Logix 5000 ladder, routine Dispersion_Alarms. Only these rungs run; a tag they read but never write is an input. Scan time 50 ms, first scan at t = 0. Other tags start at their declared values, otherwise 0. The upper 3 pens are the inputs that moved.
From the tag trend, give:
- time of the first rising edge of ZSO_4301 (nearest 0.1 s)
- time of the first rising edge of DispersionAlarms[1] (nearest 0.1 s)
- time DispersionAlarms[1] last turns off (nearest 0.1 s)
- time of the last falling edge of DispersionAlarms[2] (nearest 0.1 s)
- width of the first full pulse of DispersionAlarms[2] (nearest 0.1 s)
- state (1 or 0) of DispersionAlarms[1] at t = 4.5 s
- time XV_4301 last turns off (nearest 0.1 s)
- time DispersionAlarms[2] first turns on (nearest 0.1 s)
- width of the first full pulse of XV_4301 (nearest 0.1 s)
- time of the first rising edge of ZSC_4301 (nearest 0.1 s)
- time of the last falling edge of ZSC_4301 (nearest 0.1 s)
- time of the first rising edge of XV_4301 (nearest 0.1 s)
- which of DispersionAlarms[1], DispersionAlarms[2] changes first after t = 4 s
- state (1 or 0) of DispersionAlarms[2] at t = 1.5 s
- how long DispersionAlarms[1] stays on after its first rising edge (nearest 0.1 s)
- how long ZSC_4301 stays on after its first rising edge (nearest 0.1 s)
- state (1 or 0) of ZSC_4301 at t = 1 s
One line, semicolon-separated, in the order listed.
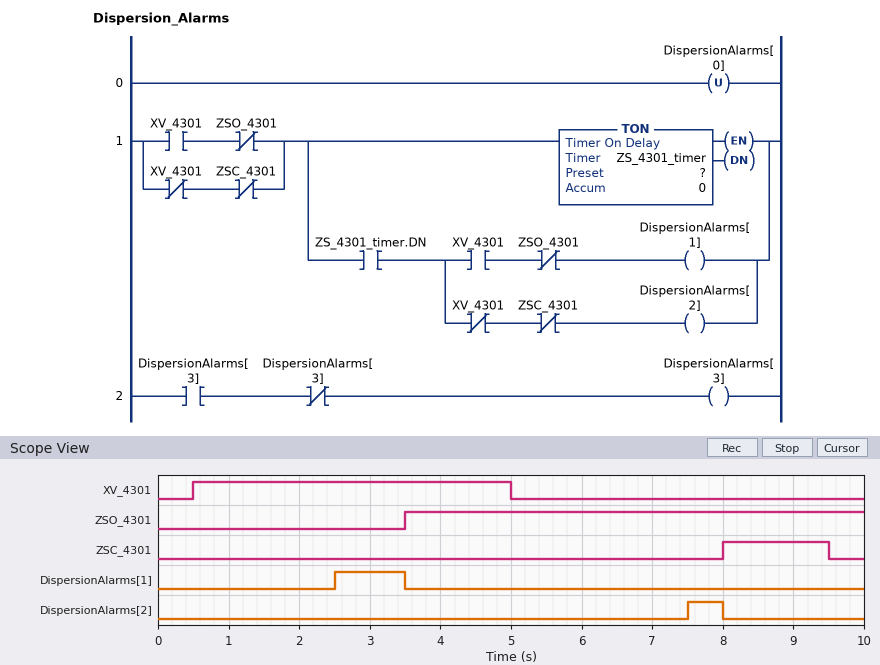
3.5 s; 2.5 s; 3.5 s; 8.0 s; 0.5 s; 0; 5.0 s; 7.5 s; 4.5 s; 8.0 s; 9.5 s; 0.5 s; DispersionAlarms[2]; 0; 1.0 s; 1.5 s; 0
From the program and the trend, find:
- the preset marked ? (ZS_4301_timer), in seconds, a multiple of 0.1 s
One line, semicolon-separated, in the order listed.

2.5 s
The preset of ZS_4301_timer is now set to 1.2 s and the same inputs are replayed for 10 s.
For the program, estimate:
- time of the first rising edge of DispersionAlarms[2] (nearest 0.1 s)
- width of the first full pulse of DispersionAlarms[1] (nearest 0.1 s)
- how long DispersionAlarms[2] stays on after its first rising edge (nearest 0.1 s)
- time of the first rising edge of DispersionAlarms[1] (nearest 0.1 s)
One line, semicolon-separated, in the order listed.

6.2 s; 2.3 s; 1.8 s; 1.2 s
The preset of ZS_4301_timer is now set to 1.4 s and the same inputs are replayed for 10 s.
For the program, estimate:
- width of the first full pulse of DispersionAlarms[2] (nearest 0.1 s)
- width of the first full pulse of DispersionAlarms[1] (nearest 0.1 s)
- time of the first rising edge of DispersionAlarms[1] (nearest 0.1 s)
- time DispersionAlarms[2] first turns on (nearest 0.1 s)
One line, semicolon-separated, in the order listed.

1.6 s; 2.1 s; 1.4 s; 6.4 s
